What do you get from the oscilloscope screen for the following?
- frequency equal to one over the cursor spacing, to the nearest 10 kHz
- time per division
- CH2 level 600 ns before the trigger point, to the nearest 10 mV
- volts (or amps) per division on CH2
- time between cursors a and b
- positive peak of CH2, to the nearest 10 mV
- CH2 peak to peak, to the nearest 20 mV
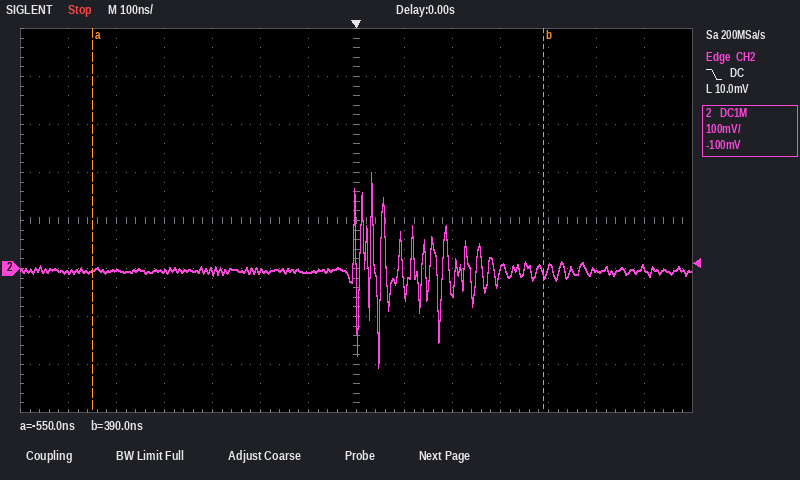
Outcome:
1.06 MHz
100 ns
-10 mV
100 mV
940 ns
200 mV
400 mV
